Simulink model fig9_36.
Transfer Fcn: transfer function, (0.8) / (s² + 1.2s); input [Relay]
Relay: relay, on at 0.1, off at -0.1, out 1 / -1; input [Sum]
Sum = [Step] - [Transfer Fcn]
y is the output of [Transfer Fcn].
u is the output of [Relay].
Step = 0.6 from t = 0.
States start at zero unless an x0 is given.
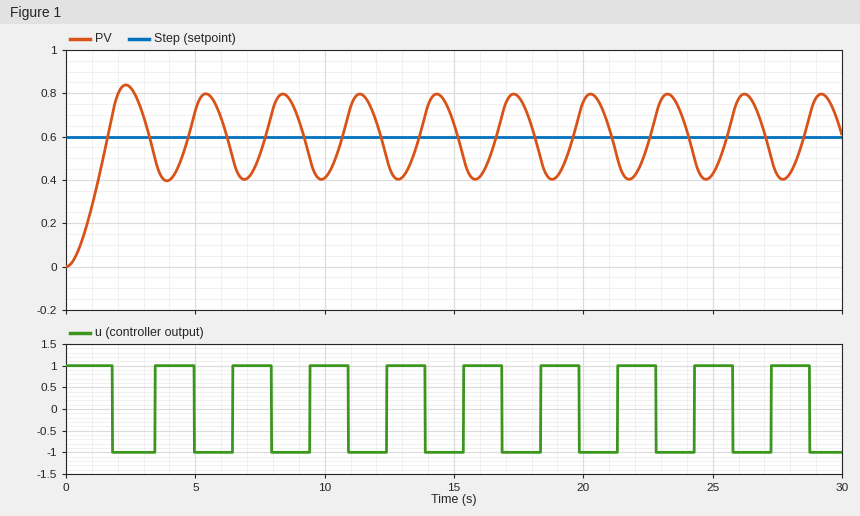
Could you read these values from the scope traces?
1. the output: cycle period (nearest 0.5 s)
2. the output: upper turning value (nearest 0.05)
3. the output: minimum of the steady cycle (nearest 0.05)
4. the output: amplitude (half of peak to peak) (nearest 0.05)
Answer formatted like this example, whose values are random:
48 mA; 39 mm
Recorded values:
3.0 s; 0.80; 0.40; 0.20
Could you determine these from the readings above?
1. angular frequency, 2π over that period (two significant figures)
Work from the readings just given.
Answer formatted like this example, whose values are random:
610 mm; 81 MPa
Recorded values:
2.1 rad/s
